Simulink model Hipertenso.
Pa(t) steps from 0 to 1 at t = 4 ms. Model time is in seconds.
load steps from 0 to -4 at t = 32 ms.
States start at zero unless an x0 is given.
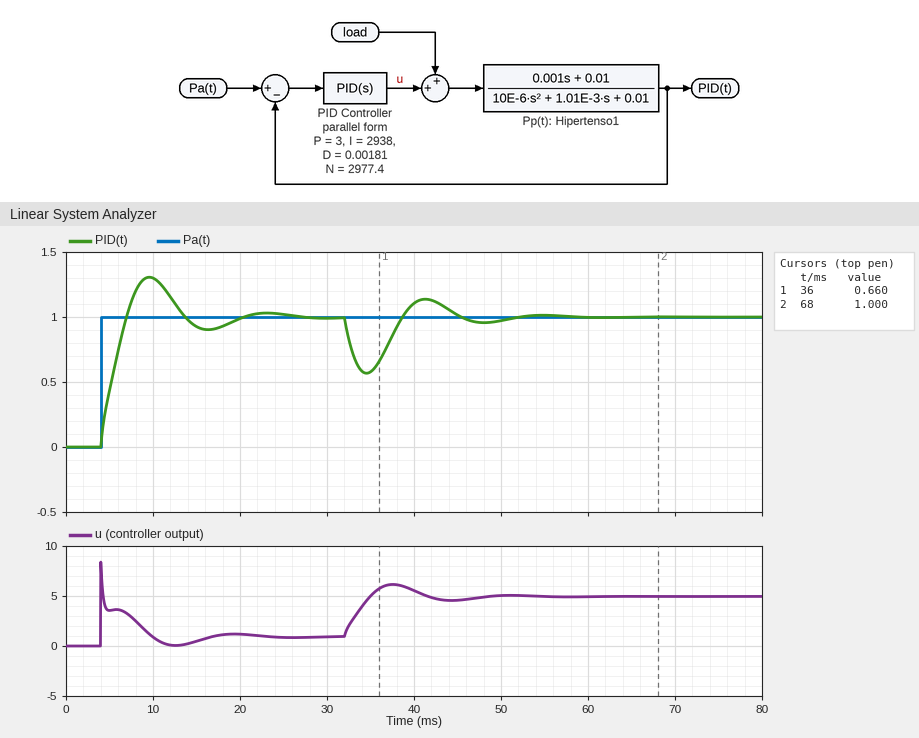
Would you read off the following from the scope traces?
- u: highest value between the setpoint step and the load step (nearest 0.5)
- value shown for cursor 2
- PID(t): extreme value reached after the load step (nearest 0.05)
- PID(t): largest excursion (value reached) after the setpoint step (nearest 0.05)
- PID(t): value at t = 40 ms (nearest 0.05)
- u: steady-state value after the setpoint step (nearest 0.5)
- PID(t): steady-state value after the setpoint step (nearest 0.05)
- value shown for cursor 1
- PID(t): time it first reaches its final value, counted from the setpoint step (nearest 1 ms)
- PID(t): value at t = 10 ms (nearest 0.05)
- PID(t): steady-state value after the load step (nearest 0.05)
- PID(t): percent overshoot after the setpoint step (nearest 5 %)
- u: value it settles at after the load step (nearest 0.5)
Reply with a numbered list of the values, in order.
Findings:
1. 8.5
2. 1.000
3. 0.55
4. 1.30
5. 1.10
6. 1.0
7. 1.00
8. 0.660
9. 3 ms
10. 1.30
11. 1.00
12. 30 %
13. 5.0
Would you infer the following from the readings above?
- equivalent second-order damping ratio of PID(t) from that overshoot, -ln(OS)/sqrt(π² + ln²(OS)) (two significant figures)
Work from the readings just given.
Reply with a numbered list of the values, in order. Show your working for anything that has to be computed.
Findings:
1. ln(0.3) = -1.204; 1.204 / sqrt(9.870 + 1.450) = 0.36
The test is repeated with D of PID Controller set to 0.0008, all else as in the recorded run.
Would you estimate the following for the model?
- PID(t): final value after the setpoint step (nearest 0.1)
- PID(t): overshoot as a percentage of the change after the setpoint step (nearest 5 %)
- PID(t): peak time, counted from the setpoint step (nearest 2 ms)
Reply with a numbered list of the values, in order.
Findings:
1. 1.0
2. 35 %
3. 6 ms
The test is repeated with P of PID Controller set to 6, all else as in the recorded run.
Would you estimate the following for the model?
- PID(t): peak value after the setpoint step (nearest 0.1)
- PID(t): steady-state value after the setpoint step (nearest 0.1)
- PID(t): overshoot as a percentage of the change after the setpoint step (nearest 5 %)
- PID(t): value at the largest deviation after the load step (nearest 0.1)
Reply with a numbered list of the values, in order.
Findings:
1. 1.2
2. 1.0
3. 15 %
4. 0.7
